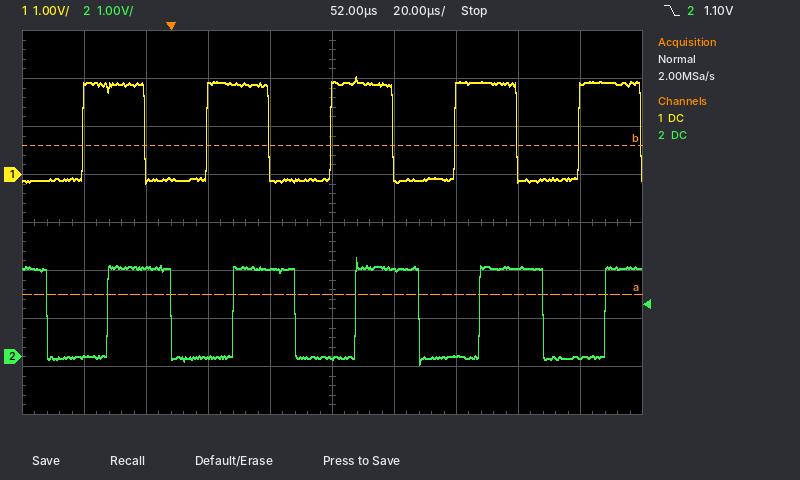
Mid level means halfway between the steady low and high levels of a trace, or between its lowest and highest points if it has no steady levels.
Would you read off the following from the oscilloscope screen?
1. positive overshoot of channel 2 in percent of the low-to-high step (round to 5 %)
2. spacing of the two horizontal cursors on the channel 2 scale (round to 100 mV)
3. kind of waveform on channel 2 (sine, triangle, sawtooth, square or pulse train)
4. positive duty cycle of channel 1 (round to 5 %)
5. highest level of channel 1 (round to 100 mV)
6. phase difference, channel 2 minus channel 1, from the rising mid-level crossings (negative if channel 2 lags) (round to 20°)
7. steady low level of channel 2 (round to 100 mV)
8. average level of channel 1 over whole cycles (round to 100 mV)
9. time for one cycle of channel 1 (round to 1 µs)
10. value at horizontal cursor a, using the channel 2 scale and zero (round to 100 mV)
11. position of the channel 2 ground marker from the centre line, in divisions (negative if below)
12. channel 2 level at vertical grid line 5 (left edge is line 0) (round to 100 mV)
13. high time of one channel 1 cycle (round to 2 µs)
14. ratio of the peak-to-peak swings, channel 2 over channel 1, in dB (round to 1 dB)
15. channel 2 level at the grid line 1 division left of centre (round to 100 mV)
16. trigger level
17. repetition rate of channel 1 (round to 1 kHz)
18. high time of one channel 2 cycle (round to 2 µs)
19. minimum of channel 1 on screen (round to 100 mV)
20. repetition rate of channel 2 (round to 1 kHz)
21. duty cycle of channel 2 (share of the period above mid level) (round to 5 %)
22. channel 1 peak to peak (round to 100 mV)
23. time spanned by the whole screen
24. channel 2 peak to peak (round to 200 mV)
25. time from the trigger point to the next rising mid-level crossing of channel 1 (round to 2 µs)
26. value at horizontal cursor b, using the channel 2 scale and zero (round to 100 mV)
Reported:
10 %
3.1 V
square
50 %
2.0 V
-80°
0.0 V
900 mV
40 µs
1.3 V
-2.8 div
0.0 V
20 µs
0 dB
1.8 V
1.10 V
25 kHz
20 µs
-200 mV
25 kHz
50 %
2.2 V
200 µs
2.2 V
12 µs
4.4 V
